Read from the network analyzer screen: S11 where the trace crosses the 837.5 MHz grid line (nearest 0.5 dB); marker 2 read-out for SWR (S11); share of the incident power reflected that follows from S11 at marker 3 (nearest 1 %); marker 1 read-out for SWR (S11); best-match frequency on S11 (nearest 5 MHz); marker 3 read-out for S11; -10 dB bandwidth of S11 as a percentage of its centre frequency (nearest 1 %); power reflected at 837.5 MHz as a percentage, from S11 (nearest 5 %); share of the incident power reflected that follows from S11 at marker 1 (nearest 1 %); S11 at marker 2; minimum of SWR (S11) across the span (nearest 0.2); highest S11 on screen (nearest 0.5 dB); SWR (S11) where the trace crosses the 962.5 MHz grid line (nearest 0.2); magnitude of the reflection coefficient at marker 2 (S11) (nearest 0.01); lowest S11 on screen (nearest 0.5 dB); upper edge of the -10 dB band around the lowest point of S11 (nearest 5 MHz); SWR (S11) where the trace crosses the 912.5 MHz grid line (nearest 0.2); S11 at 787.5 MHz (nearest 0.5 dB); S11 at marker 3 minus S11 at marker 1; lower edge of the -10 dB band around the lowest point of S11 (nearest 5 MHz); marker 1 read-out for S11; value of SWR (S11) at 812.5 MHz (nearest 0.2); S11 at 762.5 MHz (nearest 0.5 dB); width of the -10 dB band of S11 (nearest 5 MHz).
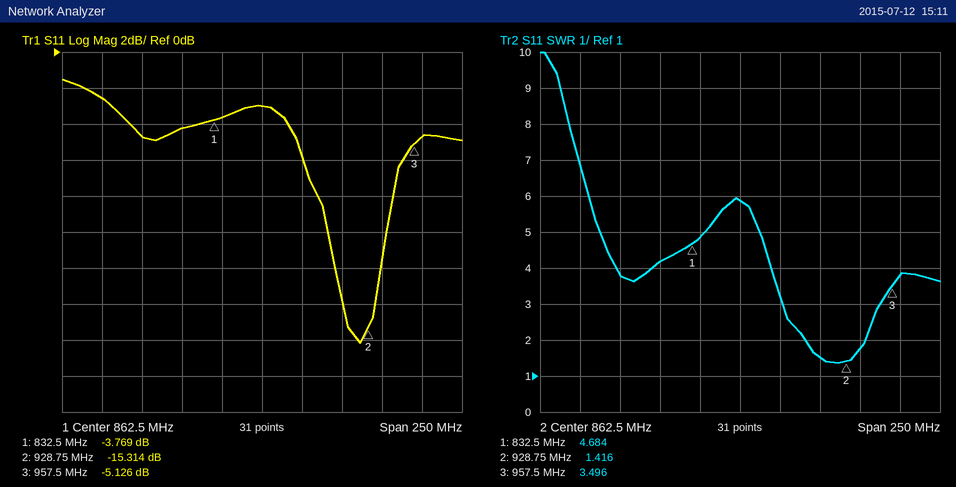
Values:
-3.5 dB
1.416
31 %
4.684
925 MHz
-5.126 dB
4 %
45 %
42 %
-15.314 dB
1.4
-1.5 dB
3.8
0.17
-16.0 dB
940 MHz
1.6
-4.5 dB
-1.357 dB
905 MHz
-3.769 dB
4.2
-2.5 dB
35 MHz
